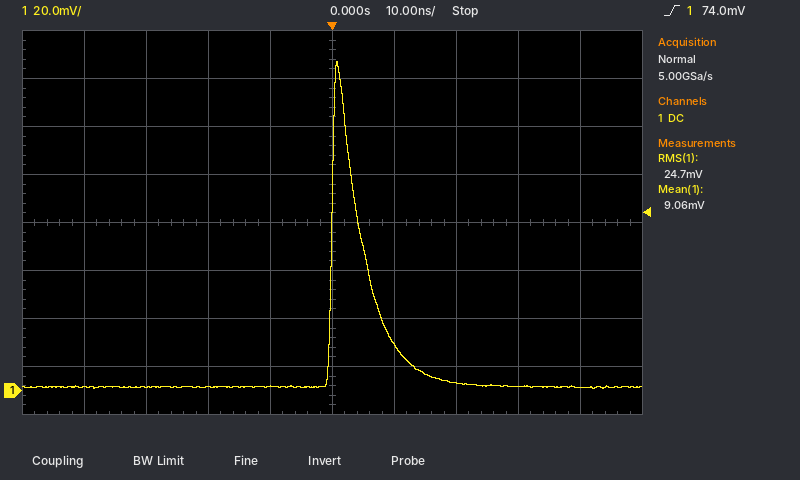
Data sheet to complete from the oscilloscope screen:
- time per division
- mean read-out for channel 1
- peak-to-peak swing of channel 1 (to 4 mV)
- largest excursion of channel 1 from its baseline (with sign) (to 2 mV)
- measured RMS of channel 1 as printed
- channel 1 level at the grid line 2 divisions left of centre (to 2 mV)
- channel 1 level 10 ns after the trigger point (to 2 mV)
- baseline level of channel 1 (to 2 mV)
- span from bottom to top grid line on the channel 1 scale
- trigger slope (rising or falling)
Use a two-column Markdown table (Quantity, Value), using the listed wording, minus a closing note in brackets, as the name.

| Quantity | Value |
|---|---|
| time per division | 10 ns |
| mean read-out for channel 1 | 9.06 mV |
| peak-to-peak swing of channel 1 | 136 mV |
| largest excursion of channel 1 from its baseline (with sign) | +136 mV |
| measured RMS of channel 1 as printed | 24.7 mV |
| channel 1 level at the grid line 2 divisions left of centre | 2 mV |
| channel 1 level 10 ns after the trigger point | 20 mV |
| baseline level of channel 1 | 2 mV |
| span from bottom to top grid line on the channel 1 scale | 160 mV |
| trigger slope | rising |
